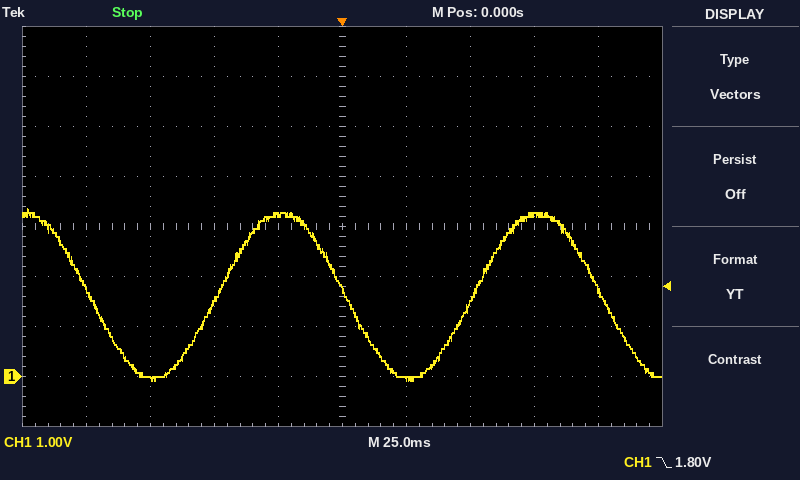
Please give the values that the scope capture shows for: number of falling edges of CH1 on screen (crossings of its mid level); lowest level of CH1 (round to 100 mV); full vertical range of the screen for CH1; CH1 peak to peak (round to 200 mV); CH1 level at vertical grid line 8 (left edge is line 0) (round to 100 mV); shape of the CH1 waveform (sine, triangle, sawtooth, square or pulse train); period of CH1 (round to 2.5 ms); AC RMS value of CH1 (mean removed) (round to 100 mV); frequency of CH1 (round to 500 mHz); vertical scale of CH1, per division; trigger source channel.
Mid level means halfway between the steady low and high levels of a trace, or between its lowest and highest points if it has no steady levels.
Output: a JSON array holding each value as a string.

["3", "-100 mV", "8 V", "3.4 V", "3.2 V", "sine", "100.0 ms", "1.2 V", "10.0 Hz", "1 V", "CH1"]
